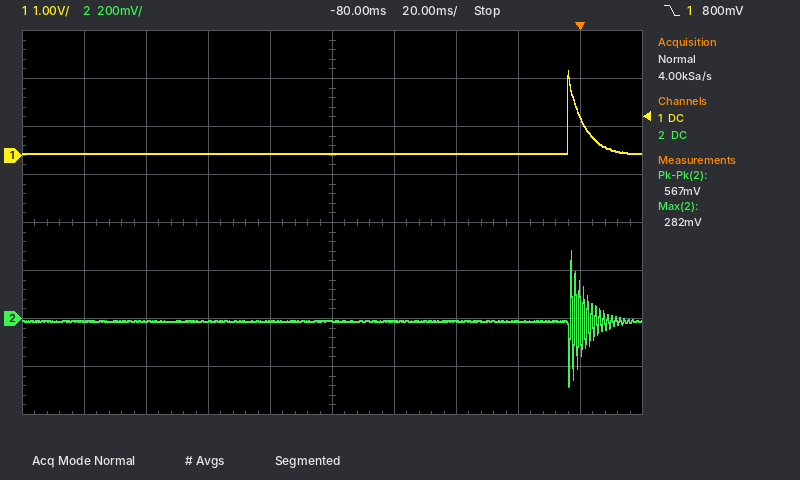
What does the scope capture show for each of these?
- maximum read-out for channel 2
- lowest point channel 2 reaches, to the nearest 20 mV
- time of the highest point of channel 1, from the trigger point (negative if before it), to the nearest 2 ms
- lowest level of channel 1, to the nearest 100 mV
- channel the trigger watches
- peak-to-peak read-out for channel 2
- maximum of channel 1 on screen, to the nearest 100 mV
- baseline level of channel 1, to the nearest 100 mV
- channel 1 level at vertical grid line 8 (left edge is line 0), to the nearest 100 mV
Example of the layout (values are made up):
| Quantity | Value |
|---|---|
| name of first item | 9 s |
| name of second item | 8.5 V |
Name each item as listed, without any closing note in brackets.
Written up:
| Quantity | Value |
|---|---|
| maximum read-out for channel 2 | 282 mV |
| lowest point channel 2 reaches, to the nearest 20 mV | -280 mV |
| time of the highest point of channel 1, from the trigger point (negative if before it), to the nearest 2 ms | -4 ms |
| lowest level of channel 1, to the nearest 100 mV | 0.0 V |
| channel the trigger watches | channel 1 |
| peak-to-peak read-out for channel 2 | 567 mV |
| maximum of channel 1 on screen, to the nearest 100 mV | 1.8 V |
| baseline level of channel 1, to the nearest 100 mV | 0.0 V |
| channel 1 level at vertical grid line 8 (left edge is line 0), to the nearest 100 mV | 0.0 V |
